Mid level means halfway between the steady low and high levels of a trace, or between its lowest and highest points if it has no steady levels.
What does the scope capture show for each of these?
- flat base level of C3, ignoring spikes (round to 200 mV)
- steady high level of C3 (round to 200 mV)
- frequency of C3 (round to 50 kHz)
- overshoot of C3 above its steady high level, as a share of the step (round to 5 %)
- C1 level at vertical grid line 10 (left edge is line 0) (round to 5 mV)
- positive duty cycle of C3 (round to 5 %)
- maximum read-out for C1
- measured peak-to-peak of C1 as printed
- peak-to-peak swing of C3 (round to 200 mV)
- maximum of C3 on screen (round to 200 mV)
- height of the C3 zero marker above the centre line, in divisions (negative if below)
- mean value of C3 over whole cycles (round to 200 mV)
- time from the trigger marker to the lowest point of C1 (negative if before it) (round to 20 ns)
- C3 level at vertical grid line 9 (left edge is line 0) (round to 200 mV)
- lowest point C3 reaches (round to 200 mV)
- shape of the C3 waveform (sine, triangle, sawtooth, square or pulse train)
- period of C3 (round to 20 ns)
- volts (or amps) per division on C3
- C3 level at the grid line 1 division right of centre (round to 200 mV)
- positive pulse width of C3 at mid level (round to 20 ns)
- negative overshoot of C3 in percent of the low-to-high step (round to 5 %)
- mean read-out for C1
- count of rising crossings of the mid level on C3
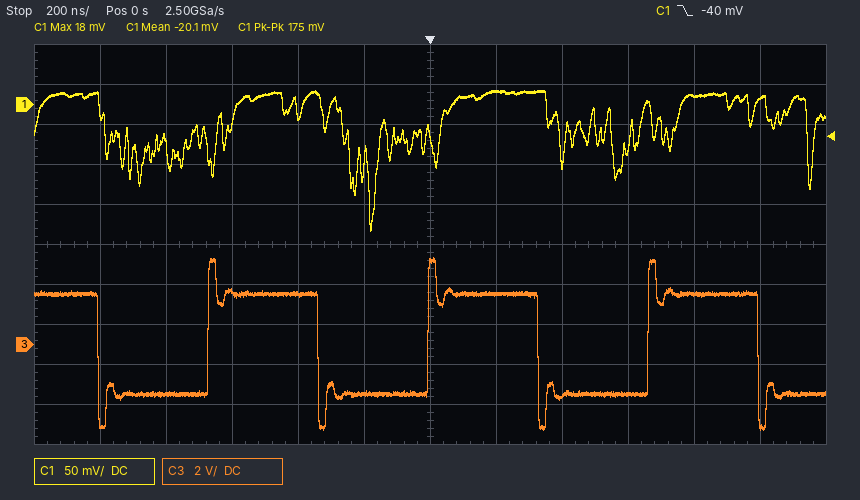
-2.4 V
2.6 V
1.50 MHz
35 %
10 mV
50 %
18 mV
175 mV
8.6 V
4.4 V
-2.5 div
0.0 V
-180 ns
-2.4 V
-4.2 V
square
660 ns
2 V
2.6 V
340 ns
35 %
-20.1 mV
3
